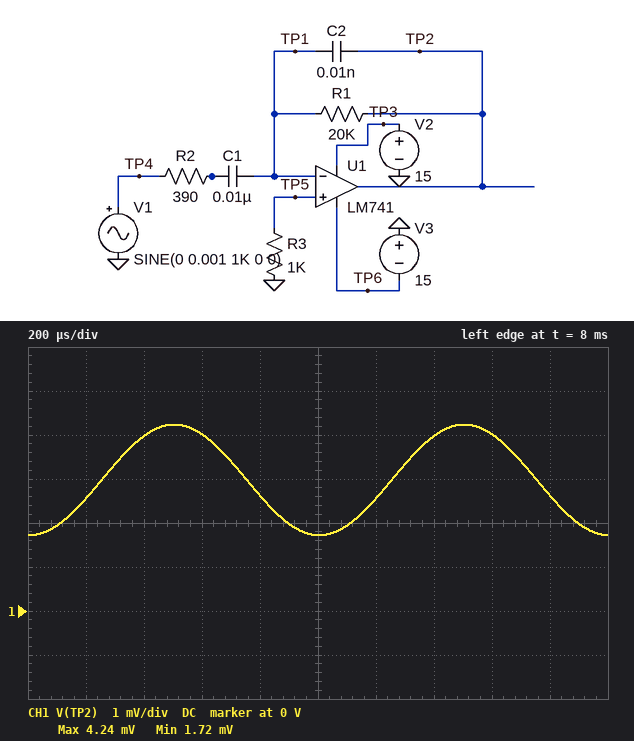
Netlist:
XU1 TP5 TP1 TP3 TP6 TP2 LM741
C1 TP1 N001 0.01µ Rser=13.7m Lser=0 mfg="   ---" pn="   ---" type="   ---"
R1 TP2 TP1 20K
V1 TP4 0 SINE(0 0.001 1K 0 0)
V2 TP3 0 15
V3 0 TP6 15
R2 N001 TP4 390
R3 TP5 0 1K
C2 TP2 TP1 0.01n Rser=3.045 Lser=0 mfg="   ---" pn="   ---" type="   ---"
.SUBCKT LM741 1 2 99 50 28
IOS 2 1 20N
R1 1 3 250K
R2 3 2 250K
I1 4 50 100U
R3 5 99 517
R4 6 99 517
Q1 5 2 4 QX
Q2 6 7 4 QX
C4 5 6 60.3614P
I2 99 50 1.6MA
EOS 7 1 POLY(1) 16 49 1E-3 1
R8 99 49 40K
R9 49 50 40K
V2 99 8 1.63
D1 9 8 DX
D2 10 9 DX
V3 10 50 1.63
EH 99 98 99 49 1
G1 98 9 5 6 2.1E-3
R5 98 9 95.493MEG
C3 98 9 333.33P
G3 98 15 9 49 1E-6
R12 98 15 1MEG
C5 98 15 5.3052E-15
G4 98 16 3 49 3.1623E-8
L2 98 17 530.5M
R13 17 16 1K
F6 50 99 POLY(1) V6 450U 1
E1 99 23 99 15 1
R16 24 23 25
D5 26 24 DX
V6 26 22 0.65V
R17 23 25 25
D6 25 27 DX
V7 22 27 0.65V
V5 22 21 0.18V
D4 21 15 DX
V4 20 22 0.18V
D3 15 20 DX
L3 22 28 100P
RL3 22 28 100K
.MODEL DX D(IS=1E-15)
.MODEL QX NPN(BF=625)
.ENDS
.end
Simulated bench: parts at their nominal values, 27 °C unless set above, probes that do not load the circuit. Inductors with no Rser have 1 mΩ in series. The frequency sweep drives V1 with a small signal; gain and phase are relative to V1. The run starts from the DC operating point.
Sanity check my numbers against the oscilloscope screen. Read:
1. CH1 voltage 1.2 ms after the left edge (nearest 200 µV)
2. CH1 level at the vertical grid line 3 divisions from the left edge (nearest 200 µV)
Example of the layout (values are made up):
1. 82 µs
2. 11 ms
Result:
1. 2.6 mV
2. 4.0 mV
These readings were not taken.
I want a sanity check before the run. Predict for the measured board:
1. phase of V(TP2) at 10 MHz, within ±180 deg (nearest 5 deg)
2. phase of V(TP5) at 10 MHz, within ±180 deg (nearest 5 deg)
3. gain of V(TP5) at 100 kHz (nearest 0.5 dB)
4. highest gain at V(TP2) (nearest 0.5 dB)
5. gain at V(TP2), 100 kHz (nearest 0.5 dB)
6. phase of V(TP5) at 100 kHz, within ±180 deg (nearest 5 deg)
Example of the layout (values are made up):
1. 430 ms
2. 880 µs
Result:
1. 55 deg
2. -25 deg
3. -49.0 dB
4. 33.5 dB
5. 20.0 dB
6. 10 deg
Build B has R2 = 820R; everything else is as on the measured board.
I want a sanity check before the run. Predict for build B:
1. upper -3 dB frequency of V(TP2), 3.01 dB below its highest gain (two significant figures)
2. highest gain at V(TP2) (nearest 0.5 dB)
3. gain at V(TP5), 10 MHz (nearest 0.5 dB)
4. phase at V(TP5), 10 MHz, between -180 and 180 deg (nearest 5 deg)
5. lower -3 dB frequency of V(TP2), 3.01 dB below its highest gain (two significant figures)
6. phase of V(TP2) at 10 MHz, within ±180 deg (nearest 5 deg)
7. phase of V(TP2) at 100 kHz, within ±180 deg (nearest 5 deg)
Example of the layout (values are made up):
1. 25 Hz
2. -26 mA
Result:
1. 53 kHz
2. 27.5 dB
3. -50.5 dB
4. -35 deg
5. 14 kHz
6. 40 deg
7. 110 deg
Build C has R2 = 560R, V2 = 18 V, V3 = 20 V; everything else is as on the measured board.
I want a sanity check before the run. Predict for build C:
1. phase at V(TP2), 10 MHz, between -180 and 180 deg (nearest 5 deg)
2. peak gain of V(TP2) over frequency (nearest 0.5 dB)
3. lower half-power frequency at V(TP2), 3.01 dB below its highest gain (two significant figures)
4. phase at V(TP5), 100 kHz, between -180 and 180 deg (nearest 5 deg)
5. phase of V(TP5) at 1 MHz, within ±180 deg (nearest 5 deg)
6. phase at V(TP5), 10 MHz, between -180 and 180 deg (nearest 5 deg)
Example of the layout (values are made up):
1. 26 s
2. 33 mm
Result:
1. 50 deg
2. 30.5 dB
3. 17 kHz
4. 15 deg
5. 0 deg
6. -30 deg
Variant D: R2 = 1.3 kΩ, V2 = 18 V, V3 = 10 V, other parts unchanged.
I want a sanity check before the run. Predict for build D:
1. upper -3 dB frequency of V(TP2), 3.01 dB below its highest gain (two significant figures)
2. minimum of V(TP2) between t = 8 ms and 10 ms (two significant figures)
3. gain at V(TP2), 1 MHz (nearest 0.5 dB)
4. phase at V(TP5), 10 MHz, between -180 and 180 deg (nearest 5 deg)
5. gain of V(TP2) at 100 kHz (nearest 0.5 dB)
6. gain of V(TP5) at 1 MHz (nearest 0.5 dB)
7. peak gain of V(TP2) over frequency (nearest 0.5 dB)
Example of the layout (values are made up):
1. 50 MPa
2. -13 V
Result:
1. 69 kHz
2. 1.6 mV
3. -1.5 dB
4. -45 deg
5. 18.0 dB
6. -50.0 dB
7. 23.5 dB
